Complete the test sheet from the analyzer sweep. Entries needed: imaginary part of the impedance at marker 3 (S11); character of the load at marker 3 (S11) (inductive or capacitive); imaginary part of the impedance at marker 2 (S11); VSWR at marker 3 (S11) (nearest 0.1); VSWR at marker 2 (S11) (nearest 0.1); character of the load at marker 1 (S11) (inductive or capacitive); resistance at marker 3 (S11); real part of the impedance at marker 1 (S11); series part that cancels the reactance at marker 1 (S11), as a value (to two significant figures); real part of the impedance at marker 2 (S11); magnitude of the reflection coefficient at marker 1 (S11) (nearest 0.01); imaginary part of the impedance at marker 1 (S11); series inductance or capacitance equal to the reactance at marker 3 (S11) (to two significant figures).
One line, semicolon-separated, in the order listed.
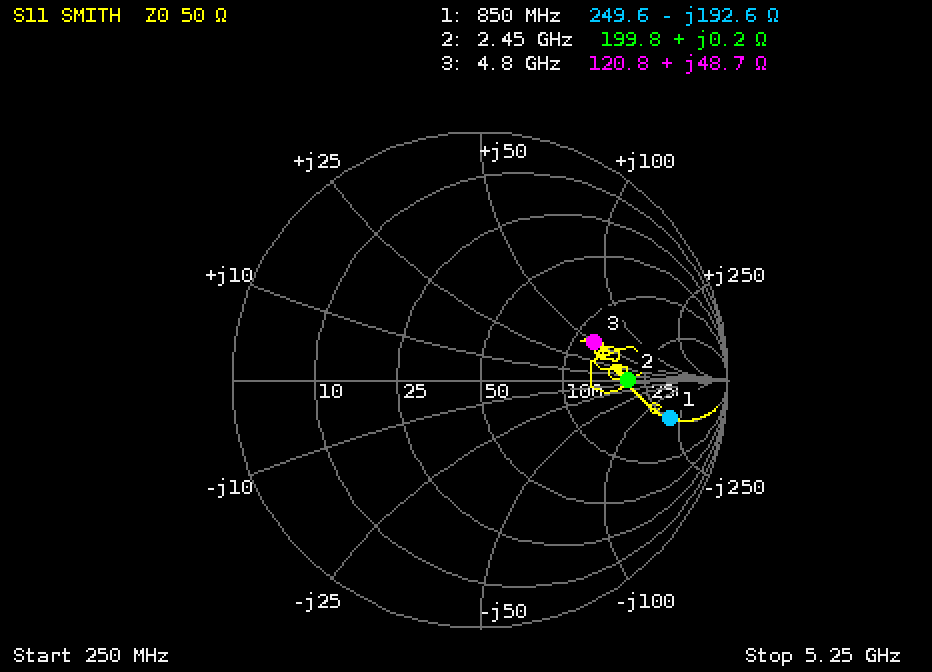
+48.7 Ω; inductive; +0.2 Ω; 2.9; 4.0; capacitive; 120.8 Ω; 249.6 Ω; 36 nH; 199.8 Ω; 0.78; -192.6 Ω; 1.6 nH
